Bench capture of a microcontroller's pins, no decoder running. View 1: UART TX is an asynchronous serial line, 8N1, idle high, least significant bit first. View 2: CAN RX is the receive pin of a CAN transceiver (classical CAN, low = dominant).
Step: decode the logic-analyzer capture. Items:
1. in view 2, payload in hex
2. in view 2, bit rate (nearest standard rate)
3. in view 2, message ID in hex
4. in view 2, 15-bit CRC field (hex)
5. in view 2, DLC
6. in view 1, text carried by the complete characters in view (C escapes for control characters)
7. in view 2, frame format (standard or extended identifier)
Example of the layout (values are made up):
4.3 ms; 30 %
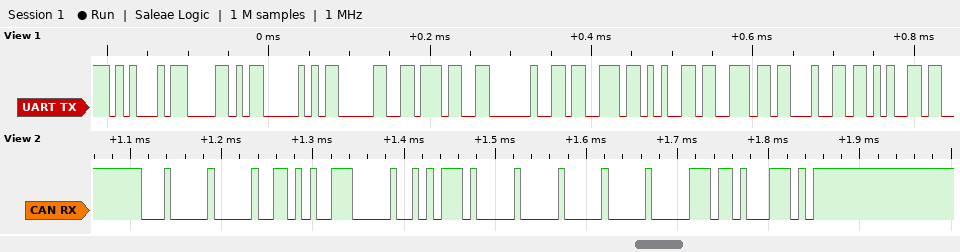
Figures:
A7 01 5D 00 00 00; 125 kbit/s; 0x100; 0x368E; 6; "EXP07 sende"; standard
